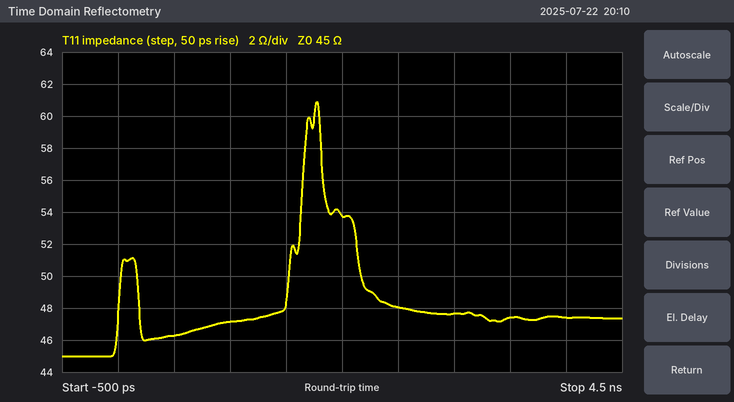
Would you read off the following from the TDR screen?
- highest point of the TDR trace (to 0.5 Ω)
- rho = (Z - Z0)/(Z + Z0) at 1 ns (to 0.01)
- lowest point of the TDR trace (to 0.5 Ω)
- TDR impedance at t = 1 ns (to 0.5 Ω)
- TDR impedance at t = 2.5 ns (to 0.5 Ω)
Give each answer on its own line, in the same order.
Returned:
61.0 Ω
+0.02
45.0 Ω
47.0 Ω
48.0 Ω
